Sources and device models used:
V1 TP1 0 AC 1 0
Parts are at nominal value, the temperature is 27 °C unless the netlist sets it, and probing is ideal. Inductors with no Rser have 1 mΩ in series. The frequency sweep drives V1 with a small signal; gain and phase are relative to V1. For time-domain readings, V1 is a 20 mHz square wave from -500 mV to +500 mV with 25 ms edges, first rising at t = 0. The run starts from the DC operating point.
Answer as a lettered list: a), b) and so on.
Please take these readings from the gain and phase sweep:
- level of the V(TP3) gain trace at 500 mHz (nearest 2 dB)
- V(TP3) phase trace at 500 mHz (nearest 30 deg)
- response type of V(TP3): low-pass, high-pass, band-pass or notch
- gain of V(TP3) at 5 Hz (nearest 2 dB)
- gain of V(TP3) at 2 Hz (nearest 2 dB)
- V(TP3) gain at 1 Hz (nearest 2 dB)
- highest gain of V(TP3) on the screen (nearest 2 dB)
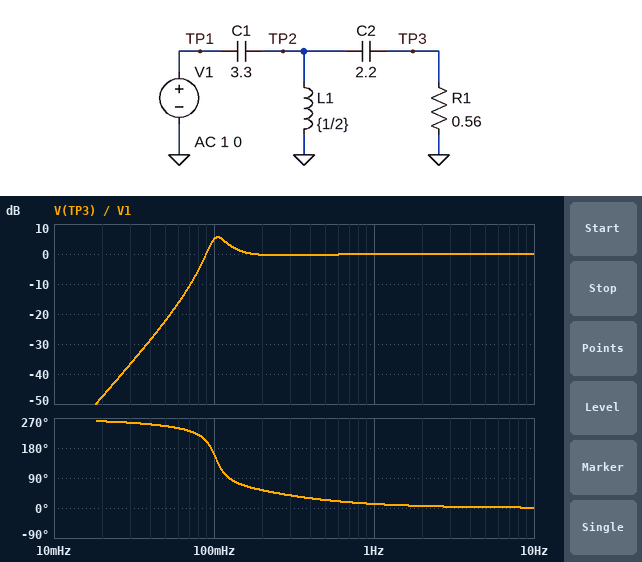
a) 0 dB
b) 30 deg
c) high-pass
d) 0 dB
e) 0 dB
f) 0 dB
g) 6 dB
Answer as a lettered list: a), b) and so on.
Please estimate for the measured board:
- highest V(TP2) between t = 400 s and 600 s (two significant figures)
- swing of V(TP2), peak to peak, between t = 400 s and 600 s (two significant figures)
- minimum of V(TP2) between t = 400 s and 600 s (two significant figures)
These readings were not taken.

a) 1.1 V
b) 2.2 V
c) -1.1 V
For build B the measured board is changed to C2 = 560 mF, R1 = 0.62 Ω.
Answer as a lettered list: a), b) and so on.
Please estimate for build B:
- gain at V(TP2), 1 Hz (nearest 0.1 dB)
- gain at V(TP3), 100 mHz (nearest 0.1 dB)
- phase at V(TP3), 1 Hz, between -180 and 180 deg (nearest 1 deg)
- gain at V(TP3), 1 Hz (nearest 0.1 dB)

a) -0.1 dB
b) -4.9 dB
c) 28 deg
d) -1.0 dB
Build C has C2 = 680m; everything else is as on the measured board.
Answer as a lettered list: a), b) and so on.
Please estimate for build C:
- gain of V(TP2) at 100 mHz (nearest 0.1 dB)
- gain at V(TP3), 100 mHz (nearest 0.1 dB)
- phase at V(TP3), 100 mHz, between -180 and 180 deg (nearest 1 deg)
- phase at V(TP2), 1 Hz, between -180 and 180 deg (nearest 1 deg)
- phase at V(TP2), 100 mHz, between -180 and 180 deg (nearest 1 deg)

a) 9.3 dB
b) -3.4 dB
c) -112 deg
d) 4 deg
e) 171 deg
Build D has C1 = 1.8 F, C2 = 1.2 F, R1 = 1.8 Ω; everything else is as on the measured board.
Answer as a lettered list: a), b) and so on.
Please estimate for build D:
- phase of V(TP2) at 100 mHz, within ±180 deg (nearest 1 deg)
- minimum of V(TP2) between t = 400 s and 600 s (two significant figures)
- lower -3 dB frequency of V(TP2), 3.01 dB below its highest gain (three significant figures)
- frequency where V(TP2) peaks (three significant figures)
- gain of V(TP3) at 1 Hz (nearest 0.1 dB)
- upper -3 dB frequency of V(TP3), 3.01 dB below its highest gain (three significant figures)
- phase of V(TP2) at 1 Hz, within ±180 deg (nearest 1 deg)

a) 168 deg
b) -960 mV
c) 143 mHz
d) 160 mHz
e) 0.2 dB
f) 188 mHz
g) 3 deg
